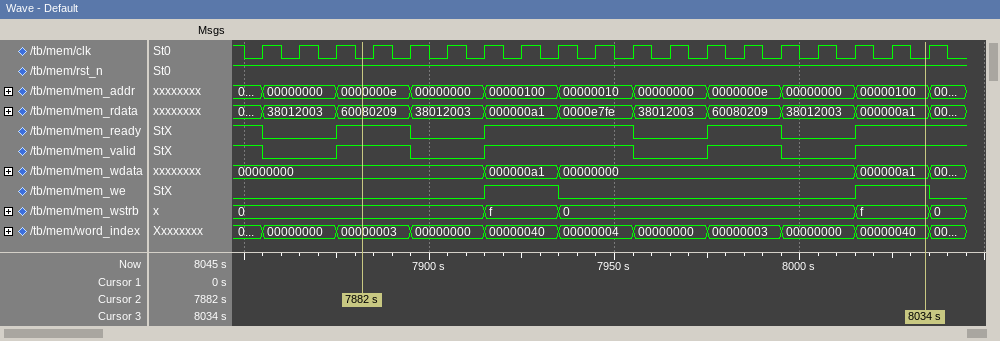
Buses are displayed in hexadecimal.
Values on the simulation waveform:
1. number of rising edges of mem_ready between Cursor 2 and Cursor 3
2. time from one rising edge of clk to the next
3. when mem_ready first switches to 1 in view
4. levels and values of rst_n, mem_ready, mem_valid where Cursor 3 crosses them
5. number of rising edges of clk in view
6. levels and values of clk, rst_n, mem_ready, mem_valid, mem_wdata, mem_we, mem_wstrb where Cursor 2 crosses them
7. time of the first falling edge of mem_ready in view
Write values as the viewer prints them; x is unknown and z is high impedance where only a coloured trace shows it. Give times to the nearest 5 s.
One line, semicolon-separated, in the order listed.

3; 10 s; 7875 s; rst_n=1, mem_ready=1, mem_valid=1; 19; clk=0, rst_n=1, mem_ready=1, mem_valid=1, mem_wdata=00000000, mem_we=0, mem_wstrb=0; 7855 s
